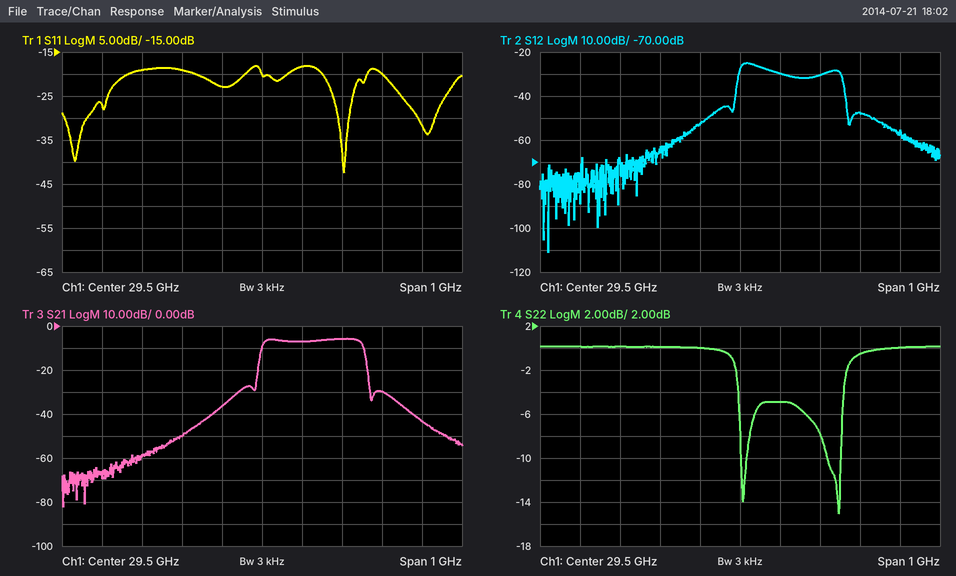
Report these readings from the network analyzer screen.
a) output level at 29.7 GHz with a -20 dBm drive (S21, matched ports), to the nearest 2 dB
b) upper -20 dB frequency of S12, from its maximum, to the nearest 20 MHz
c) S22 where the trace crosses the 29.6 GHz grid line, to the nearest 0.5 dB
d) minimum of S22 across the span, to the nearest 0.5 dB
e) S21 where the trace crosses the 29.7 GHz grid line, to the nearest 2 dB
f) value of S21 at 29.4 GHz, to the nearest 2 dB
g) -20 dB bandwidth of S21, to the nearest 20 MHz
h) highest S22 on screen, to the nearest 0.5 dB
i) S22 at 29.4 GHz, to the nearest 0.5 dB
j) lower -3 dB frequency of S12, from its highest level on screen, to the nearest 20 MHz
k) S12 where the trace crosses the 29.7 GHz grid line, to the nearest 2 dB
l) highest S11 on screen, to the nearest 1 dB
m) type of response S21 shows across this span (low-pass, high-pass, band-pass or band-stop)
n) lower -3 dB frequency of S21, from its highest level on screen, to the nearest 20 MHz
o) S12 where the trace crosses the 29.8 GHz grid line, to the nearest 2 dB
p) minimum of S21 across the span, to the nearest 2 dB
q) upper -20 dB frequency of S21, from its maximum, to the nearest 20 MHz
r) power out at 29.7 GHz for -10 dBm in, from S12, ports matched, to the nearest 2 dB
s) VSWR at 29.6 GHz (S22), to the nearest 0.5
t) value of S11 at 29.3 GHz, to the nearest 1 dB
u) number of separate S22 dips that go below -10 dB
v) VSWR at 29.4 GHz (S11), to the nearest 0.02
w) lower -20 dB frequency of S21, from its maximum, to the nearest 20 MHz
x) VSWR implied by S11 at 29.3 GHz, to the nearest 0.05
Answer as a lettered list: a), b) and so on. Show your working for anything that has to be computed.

a) -20 dBm + (-6 dB) = -26 dBm
b) 29.76 GHz
c) -5.0 dB
d) -15.0 dB
e) -6 dB
f) -36 dB
g) 29.76 GHz − 29.48 GHz = 280 MHz
h) 0.0 dB
i) 0.0 dB
j) 29.50 GHz
k) -30 dB
l) -18 dB
m) band-pass
n) 29.50 GHz
o) -48 dB
p) -82 dB
q) 29.76 GHz
r) -10 dBm + (-30 dB) = -40 dBm
s) |Γ| = 10^(-5/20) = 0.5623; VSWR = (1 + 0.5623)/(1 − 0.5623) ≈ 3.57, so 3.5 to the nearest 0.5
t) -19 dB
u) 2
v) |Γ| = 10^(-23/20) = 0.0708; VSWR = (1 + 0.0708)/(1 − 0.0708) ≈ 1.15, so 1.16 to the nearest 0.02
w) 29.48 GHz
x) |Γ| = 10^(-19/20) = 0.1122; VSWR = (1 + 0.1122)/(1 − 0.1122) ≈ 1.25
